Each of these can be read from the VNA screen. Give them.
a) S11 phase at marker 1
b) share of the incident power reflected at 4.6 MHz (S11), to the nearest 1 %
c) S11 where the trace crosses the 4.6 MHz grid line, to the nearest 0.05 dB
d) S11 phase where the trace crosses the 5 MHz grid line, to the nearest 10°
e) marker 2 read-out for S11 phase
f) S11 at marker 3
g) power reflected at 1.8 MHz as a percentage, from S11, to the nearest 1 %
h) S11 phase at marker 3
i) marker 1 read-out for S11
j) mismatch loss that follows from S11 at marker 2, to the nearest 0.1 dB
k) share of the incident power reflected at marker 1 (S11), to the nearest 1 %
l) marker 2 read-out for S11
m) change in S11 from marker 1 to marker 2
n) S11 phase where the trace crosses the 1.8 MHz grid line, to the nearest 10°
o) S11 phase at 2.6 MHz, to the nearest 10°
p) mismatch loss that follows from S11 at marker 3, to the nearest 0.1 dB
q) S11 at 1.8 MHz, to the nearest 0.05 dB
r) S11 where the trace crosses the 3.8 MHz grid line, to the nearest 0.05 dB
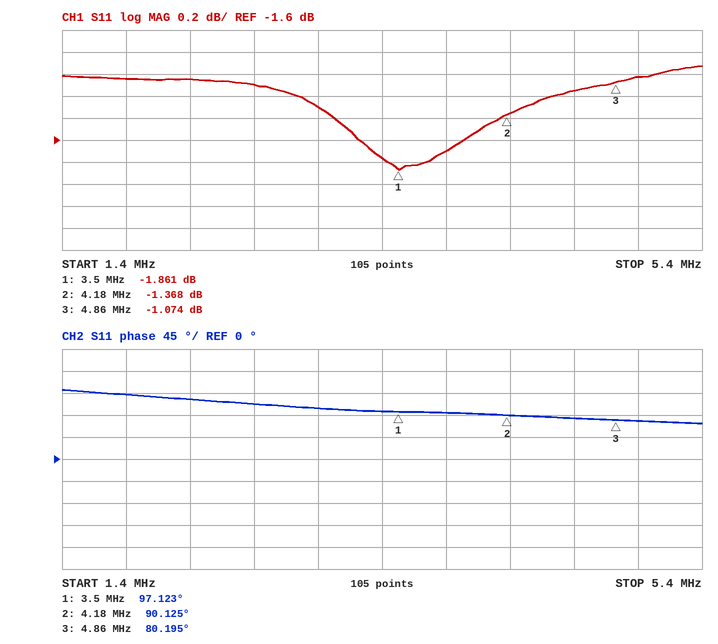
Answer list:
97.123°
77 %
-1.15 dB
80°
90.125°
-1.074 dB
79 %
80.195°
-1.861 dB
5.7 dB
65 %
-1.368 dB
0.493 dB
130°
110°
6.6 dB
-1.05 dB
-1.70 dB
